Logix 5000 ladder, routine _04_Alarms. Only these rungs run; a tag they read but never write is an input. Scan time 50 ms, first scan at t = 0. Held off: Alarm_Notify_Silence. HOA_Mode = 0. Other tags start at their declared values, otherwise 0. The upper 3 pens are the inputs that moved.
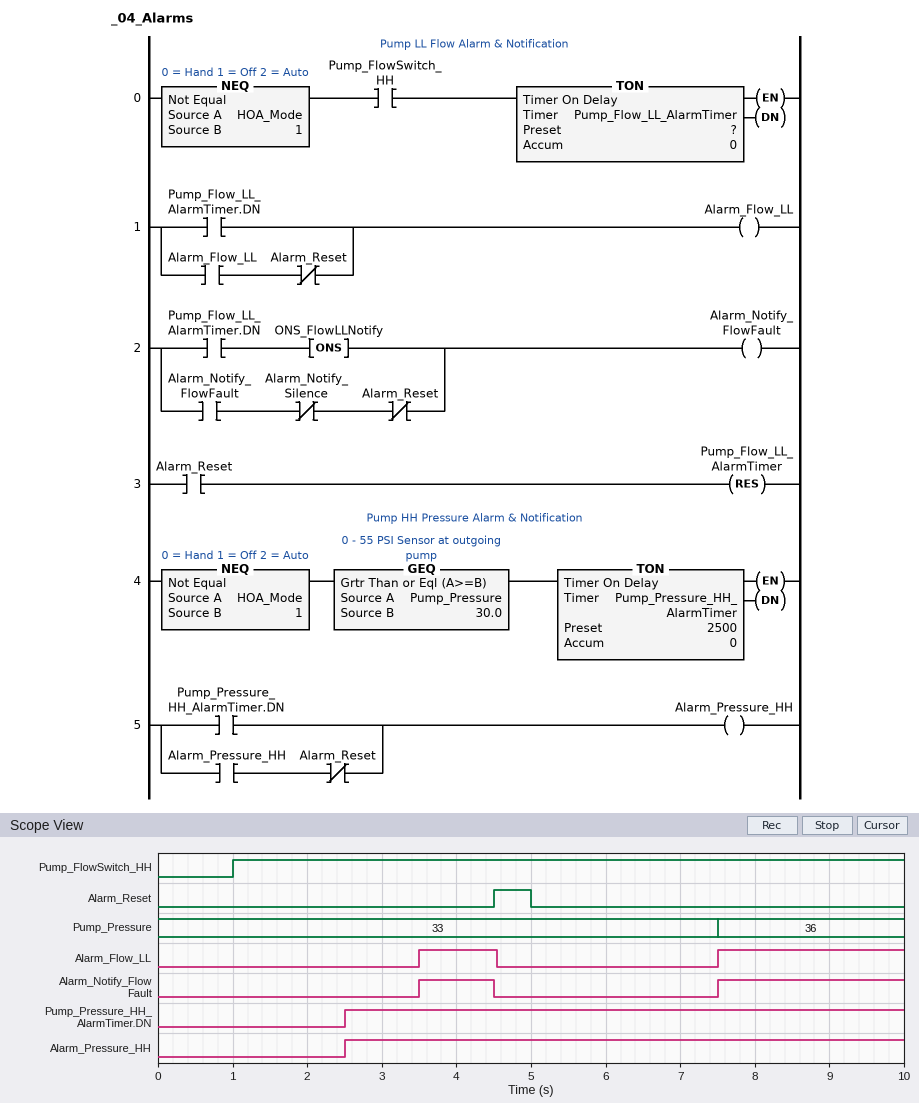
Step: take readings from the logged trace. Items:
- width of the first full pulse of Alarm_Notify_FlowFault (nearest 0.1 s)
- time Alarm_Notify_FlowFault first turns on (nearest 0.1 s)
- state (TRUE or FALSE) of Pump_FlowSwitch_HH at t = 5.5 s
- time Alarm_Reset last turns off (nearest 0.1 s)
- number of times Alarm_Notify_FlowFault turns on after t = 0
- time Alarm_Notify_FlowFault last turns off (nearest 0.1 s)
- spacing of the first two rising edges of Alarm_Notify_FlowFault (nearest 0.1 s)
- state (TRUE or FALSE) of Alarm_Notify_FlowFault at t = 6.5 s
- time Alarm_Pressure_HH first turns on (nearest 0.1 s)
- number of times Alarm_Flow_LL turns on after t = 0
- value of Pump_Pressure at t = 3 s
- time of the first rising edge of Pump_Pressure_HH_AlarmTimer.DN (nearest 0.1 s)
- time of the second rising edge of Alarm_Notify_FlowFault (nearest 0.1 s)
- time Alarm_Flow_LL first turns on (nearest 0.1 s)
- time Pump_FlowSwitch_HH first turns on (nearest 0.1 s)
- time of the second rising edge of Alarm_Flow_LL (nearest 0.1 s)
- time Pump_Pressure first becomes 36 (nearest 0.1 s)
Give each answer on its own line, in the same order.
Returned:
1.0 s
3.5 s
TRUE
5.0 s
2
4.5 s
4.0 s
FALSE
2.5 s
2
33
2.5 s
7.5 s
3.5 s
1.0 s
7.5 s
7.5 s
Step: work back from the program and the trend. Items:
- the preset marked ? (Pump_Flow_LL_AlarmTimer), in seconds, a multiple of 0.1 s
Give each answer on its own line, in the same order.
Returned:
2.5 s
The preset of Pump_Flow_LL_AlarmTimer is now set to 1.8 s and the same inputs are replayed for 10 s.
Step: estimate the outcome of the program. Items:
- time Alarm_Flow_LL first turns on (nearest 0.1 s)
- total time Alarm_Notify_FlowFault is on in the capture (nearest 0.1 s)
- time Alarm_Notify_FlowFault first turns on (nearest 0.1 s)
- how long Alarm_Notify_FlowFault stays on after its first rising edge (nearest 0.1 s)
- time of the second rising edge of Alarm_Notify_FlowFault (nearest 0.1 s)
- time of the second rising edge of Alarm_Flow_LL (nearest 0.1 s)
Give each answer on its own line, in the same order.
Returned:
2.8 s
4.9 s
2.8 s
1.7 s
6.8 s
6.8 s
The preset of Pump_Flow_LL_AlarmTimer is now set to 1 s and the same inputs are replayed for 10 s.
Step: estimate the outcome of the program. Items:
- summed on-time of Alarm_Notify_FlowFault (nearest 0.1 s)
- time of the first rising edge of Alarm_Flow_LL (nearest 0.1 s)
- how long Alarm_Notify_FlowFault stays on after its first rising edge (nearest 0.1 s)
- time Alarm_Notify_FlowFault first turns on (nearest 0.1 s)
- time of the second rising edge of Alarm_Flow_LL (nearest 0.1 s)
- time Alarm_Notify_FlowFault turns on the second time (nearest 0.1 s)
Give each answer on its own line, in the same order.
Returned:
6.5 s
2.0 s
2.5 s
2.0 s
6.0 s
6.0 s
